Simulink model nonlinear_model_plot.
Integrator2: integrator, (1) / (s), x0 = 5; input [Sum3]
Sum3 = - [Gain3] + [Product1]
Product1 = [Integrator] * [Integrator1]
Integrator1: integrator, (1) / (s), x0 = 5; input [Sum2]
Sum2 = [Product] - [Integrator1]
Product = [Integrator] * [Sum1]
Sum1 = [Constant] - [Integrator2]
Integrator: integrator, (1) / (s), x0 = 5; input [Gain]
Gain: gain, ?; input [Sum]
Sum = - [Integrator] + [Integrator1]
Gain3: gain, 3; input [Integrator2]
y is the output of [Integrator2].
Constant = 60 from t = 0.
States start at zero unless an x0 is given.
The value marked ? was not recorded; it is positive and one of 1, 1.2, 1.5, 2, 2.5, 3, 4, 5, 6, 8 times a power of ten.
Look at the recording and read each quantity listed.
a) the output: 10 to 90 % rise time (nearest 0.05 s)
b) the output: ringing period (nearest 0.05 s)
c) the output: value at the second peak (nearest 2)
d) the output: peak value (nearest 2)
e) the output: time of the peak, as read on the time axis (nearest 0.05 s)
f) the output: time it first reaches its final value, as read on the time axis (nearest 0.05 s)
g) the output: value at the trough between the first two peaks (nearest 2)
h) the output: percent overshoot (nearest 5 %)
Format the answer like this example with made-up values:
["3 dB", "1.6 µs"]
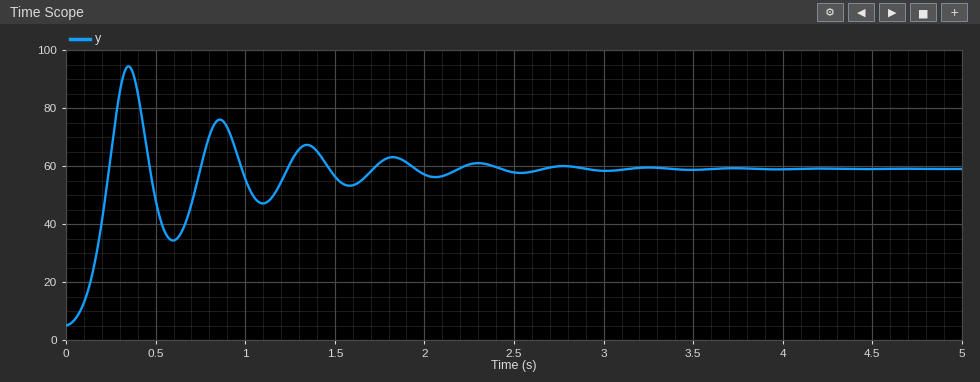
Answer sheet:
["0.15 s", "0.50 s", "76", "94", "0.35 s", "0.25 s", "34", "65 %"]
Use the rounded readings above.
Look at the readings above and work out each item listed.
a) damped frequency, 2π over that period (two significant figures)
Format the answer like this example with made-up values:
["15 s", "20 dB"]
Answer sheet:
["13 rad/s"]
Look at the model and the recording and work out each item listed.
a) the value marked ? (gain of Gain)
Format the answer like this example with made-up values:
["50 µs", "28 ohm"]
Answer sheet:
["1"]
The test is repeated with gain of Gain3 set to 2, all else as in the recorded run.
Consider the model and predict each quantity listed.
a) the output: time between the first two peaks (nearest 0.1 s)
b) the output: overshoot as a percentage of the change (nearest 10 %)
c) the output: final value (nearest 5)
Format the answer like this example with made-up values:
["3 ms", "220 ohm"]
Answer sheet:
["0.6 s", "70 %", "60"]
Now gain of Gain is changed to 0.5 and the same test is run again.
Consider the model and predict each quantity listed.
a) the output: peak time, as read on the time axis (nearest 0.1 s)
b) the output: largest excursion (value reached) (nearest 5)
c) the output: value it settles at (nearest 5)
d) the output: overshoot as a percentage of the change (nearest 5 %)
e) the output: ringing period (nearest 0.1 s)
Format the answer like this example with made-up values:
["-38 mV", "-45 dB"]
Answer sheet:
["0.4 s", "90", "60", "55 %", "0.6 s"]
